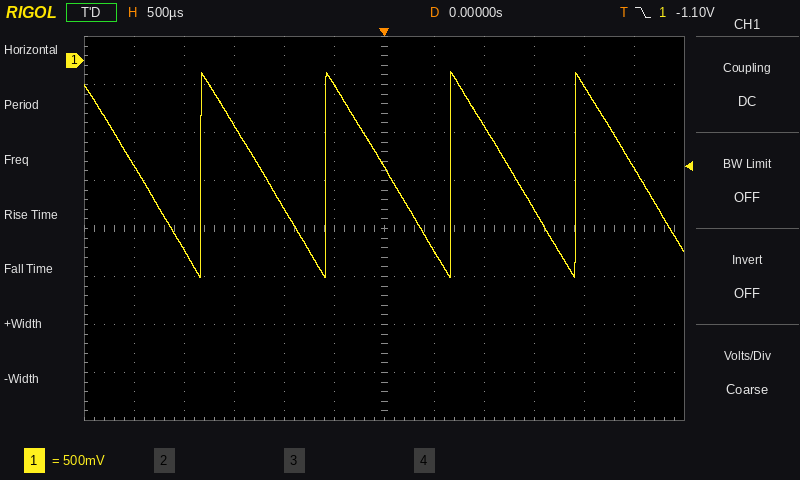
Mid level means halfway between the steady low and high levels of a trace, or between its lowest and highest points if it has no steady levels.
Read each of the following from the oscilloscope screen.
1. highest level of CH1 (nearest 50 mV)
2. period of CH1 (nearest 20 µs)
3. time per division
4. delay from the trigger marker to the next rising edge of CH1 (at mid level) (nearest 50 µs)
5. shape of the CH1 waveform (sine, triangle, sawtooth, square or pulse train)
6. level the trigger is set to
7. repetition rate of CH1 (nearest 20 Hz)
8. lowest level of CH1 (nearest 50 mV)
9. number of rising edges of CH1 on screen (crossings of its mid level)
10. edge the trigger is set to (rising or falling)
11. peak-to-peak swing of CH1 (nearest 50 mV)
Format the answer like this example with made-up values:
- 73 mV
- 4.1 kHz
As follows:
- -100 mV
- 1.24 ms
- 500 µs
- 650 µs
- sawtooth
- -1.10 V
- 800 Hz
- -2.25 V
- 4
- falling
- 2.15 V
